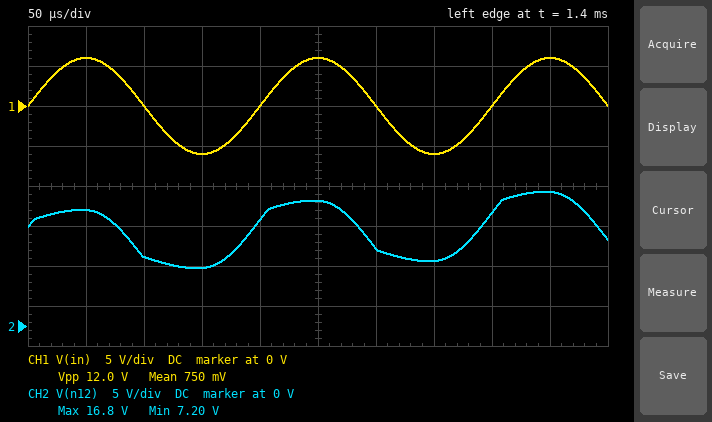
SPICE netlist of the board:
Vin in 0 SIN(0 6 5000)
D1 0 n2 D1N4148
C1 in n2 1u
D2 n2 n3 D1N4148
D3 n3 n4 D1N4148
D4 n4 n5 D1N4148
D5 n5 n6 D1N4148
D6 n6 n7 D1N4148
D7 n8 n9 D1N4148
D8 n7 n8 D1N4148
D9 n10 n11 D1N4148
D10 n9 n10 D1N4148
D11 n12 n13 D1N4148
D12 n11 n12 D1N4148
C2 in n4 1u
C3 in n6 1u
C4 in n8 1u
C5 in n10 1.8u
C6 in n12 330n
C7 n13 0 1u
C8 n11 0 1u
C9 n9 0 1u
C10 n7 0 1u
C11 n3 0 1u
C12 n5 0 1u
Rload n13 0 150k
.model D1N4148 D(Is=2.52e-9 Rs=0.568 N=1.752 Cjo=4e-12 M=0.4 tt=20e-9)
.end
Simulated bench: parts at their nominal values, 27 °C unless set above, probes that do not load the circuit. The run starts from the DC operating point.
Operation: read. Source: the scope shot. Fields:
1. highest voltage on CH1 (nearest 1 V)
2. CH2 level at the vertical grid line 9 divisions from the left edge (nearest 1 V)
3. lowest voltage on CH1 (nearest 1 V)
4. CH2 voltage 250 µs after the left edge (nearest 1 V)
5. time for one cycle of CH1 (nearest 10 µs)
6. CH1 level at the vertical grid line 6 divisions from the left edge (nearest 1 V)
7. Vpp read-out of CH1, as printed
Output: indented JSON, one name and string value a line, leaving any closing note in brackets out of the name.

{
  "highest voltage on CH1": "6 V",
  "CH2 level at the vertical grid line 9 divisions from the left edge": "17 V",
  "lowest voltage on CH1": "-6 V",
  "CH2 voltage 250 µs after the left edge": "16 V",
  "time for one cycle of CH1": "200 µs",
  "CH1 level at the vertical grid line 6 divisions from the left edge": "0 V",
  "Vpp read-out of CH1, as printed": "12.0 V"
}
